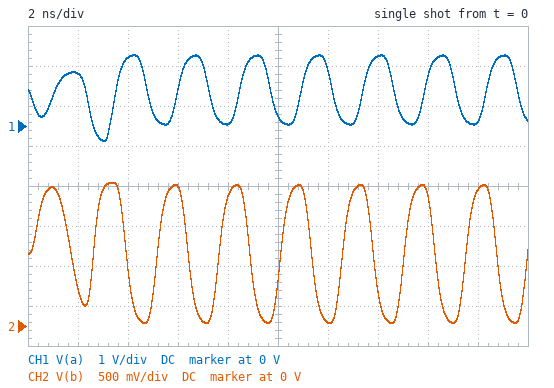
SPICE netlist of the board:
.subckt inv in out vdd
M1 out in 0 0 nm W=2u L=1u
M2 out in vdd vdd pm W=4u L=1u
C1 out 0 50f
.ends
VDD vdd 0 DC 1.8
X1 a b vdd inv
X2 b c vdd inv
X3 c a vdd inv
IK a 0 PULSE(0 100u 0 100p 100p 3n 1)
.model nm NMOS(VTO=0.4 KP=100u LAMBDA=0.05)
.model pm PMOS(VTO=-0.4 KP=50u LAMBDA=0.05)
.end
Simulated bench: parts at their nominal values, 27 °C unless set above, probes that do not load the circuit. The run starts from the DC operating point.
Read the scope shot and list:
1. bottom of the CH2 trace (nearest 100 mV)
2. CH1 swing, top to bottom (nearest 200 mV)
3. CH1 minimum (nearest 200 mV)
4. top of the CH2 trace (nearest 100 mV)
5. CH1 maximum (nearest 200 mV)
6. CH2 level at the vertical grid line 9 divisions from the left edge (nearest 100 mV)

0 V
2.2 V
-400 mV
1.8 V
1.8 V
1.7 V
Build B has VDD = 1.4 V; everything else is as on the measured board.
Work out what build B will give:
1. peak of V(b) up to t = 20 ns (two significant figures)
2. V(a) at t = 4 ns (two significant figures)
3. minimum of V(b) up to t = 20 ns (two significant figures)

1.4 V
1.2 V
16 mV
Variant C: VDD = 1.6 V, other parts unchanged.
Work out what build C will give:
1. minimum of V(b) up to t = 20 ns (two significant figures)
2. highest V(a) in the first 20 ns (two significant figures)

26 mV
1.6 V
